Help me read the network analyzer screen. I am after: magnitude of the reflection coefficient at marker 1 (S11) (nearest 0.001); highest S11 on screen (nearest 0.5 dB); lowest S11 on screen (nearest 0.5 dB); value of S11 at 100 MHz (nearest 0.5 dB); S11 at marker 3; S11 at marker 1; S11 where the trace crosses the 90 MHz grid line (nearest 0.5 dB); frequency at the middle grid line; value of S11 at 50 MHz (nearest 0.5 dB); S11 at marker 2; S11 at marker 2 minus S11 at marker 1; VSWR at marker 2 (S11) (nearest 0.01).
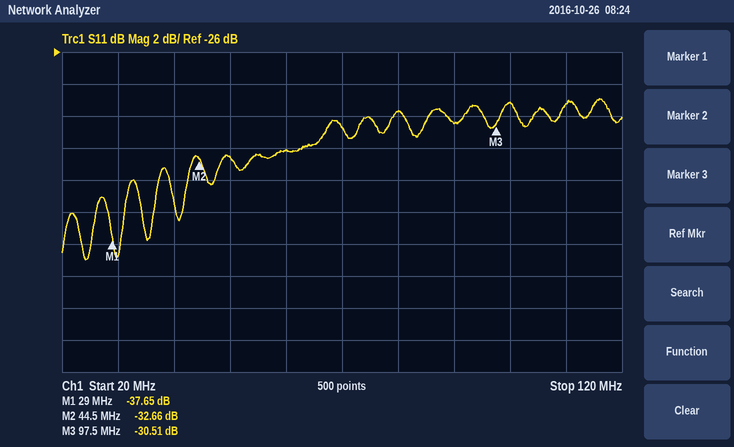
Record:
0.013
-29.0 dB
-39.0 dB
-29.0 dB
-30.51 dB
-37.65 dB
-30.5 dB
70 MHz
-32.5 dB
-32.66 dB
4.99 dB
1.05
